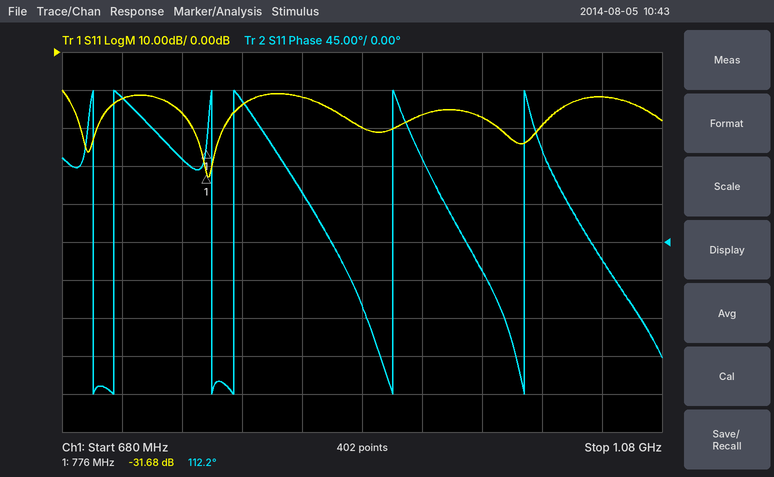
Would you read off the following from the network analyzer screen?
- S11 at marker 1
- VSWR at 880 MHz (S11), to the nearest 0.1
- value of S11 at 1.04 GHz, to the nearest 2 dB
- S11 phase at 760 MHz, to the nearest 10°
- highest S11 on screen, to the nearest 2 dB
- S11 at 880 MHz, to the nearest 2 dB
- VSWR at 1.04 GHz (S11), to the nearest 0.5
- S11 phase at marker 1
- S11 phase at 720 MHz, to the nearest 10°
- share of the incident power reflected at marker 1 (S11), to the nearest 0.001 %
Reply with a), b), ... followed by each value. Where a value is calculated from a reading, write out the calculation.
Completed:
a) -31.68 dB
b) |Γ| = 10^(-20/20) = 0.1000; VSWR = (1 + 0.1000)/(1 − 0.1000) ≈ 1.2
c) -12 dB
d) 100°
e) -10 dB
f) -20 dB
g) |Γ| = 10^(-12/20) = 0.2512; VSWR = (1 + 0.2512)/(1 − 0.2512) ≈ 1.67, so 1.5 to the nearest 0.5
h) 112.2°
i) 170°
j) 10^(-31.68/10) ≈ 0.068 %
